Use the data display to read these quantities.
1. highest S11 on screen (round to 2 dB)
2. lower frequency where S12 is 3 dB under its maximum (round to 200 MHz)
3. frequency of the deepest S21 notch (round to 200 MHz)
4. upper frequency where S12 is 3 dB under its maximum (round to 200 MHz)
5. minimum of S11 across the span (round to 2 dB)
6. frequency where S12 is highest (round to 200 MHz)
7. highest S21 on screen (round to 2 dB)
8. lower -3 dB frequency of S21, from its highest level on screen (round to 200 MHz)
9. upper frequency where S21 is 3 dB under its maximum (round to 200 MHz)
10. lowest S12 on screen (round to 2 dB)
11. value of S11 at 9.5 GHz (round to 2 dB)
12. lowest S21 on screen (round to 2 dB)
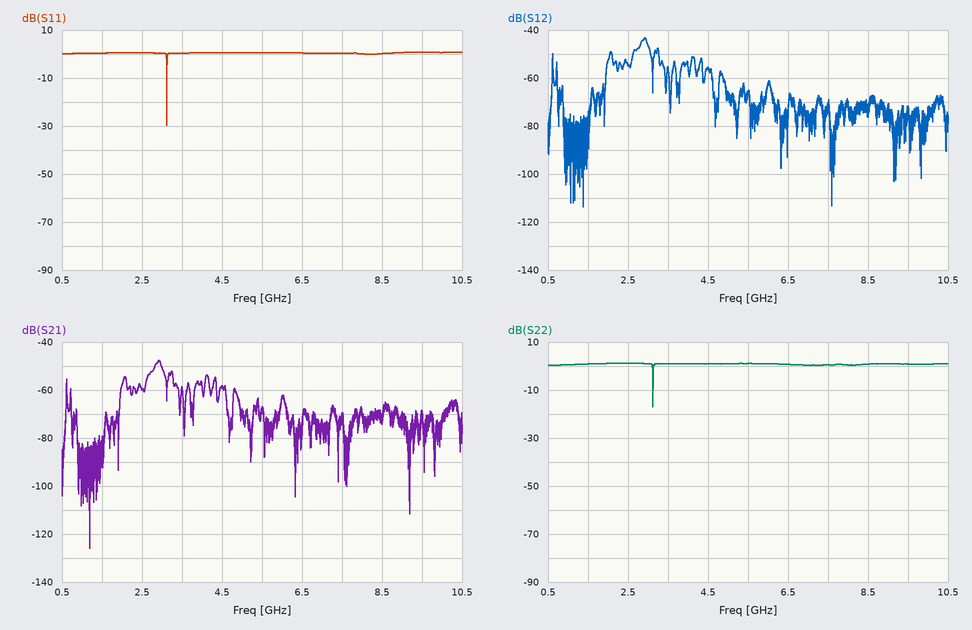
0 dB
2.8 GHz
1.2 GHz
3.0 GHz
-30 dB
3.0 GHz
-48 dB
2.8 GHz
3.0 GHz
-114 dB
0 dB
-126 dB
